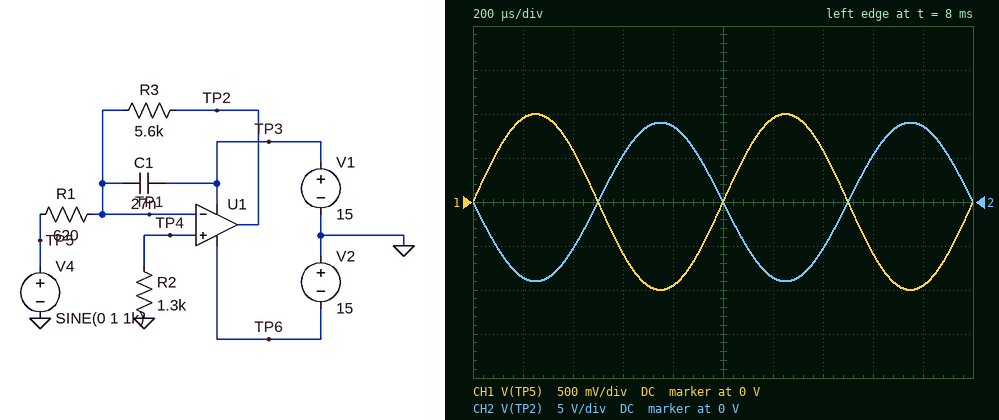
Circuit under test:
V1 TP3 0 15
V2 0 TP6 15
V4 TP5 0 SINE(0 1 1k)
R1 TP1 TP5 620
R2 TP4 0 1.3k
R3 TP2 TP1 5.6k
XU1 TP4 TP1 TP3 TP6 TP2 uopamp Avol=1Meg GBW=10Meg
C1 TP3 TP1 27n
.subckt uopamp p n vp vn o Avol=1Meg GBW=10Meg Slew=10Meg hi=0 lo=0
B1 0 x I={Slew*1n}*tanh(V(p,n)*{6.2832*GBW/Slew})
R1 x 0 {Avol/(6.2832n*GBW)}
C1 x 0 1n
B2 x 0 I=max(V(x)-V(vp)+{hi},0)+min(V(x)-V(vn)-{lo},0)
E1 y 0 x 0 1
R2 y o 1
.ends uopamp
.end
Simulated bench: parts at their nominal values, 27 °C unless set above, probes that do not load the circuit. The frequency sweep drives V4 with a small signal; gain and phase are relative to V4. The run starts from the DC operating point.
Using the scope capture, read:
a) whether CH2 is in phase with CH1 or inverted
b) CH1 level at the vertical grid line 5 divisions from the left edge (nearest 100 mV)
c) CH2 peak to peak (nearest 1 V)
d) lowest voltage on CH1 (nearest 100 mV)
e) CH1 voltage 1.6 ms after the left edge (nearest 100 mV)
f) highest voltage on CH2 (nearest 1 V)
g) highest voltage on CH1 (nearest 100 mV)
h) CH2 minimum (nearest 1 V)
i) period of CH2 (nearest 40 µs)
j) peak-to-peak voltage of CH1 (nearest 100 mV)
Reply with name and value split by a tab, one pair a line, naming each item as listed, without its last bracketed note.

whether CH2 is in phase with CH1 or inverted	inverted
CH1 level at the vertical grid line 5 divisions from the left edge	0 V
CH2 peak to peak	18 V
lowest voltage on CH1	-1.0 V
CH1 voltage 1.6 ms after the left edge	-600 mV
highest voltage on CH2	9 V
highest voltage on CH1	1.0 V
CH2 minimum	-9 V
period of CH2	1.00 ms
peak-to-peak voltage of CH1	2.0 V
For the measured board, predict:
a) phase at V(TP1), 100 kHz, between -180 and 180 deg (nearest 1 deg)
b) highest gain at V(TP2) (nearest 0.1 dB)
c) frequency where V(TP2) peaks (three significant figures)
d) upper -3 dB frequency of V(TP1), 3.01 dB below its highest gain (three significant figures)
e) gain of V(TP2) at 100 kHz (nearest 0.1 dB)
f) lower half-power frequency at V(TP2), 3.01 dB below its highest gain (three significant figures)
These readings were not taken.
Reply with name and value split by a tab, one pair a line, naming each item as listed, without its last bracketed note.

phase at V(TP1), 100 kHz, between -180 and 180 deg	26 deg
highest gain at V(TP2)	38.9 dB
frequency where V(TP2) peaks	102 kHz
upper -3 dB frequency of V(TP1), 3.01 dB below its highest gain	108 kHz
gain of V(TP2) at 100 kHz	38.1 dB
lower half-power frequency at V(TP2), 3.01 dB below its highest gain	96.9 kHz
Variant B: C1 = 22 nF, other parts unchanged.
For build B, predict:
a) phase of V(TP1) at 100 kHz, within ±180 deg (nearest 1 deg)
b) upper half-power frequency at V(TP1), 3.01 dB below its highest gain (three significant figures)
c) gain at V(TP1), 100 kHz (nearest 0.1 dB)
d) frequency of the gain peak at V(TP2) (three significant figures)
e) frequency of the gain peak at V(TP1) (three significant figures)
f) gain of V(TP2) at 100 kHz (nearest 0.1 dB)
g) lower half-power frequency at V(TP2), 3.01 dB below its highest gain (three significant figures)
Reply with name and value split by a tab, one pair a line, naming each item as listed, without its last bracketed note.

phase of V(TP1) at 100 kHz, within ±180 deg	66 deg
upper half-power frequency at V(TP1), 3.01 dB below its highest gain	120 kHz
gain at V(TP1), 100 kHz	-8.7 dB
frequency of the gain peak at V(TP2)	113 kHz
frequency of the gain peak at V(TP1)	114 kHz
gain of V(TP2) at 100 kHz	31.3 dB
lower half-power frequency at V(TP2), 3.01 dB below its highest gain	107 kHz
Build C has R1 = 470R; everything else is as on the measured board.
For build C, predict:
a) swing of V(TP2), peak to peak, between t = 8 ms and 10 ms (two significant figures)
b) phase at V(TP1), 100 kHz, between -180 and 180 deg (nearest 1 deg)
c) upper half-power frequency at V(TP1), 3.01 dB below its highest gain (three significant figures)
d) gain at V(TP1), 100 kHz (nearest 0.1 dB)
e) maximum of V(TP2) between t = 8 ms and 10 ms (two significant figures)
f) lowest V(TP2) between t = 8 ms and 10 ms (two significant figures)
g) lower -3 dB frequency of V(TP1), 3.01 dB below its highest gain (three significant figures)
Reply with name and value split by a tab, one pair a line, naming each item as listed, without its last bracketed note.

swing of V(TP2), peak to peak, between t = 8 ms and 10 ms	24 V
phase at V(TP1), 100 kHz, between -180 and 180 deg	21 deg
upper half-power frequency at V(TP1), 3.01 dB below its highest gain	110 kHz
gain at V(TP1), 100 kHz	-1.3 dB
maximum of V(TP2) between t = 8 ms and 10 ms	12 V
lowest V(TP2) between t = 8 ms and 10 ms	-12 V
lower -3 dB frequency of V(TP1), 3.01 dB below its highest gain	96.0 kHz
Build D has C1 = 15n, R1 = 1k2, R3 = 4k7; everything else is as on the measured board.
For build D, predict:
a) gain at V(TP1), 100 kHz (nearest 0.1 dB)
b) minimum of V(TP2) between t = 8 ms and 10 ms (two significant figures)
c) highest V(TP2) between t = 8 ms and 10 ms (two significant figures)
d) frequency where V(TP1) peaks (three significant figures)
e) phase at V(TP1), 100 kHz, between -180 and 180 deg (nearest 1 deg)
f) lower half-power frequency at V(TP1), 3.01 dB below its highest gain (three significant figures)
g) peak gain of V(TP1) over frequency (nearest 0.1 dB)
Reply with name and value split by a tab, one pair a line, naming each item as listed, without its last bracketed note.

gain at V(TP1), 100 kHz	-23.1 dB
minimum of V(TP2) between t = 8 ms and 10 ms	-3.9 V
highest V(TP2) between t = 8 ms and 10 ms	3.9 V
frequency where V(TP1) peaks	150 kHz
phase at V(TP1), 100 kHz, between -180 and 180 deg	85 deg
lower half-power frequency at V(TP1), 3.01 dB below its highest gain	145 kHz
peak gain of V(TP1) over frequency	-2.0 dB
